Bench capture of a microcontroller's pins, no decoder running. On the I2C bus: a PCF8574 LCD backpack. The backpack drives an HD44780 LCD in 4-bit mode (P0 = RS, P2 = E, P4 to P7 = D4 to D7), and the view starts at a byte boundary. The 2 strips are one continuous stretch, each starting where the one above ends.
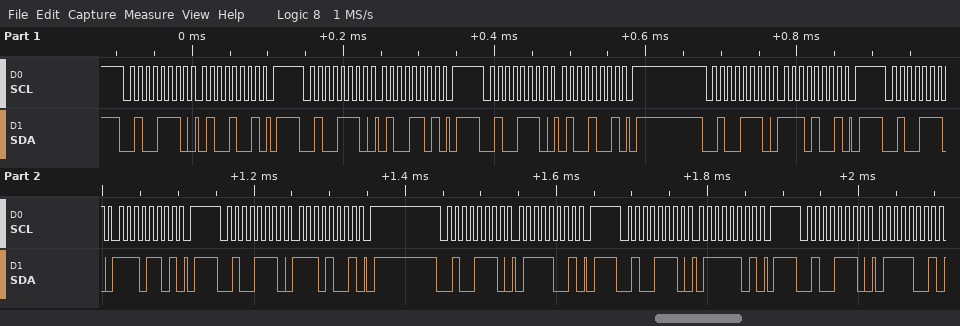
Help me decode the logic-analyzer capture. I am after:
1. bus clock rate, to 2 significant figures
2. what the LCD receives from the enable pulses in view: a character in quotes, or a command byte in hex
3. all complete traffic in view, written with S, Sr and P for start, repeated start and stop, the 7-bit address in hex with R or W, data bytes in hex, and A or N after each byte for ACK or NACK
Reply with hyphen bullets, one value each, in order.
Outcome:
- 100 kHz
- 'N'
- S 27W A 49 A P S 27W A 4D A P S 27W A 49 A P S 27W A E9 A P S 27W A ED A P S 27W A E9 A P S 27W A 79 A P S 27W A 7D A P S 27W A 79 A
